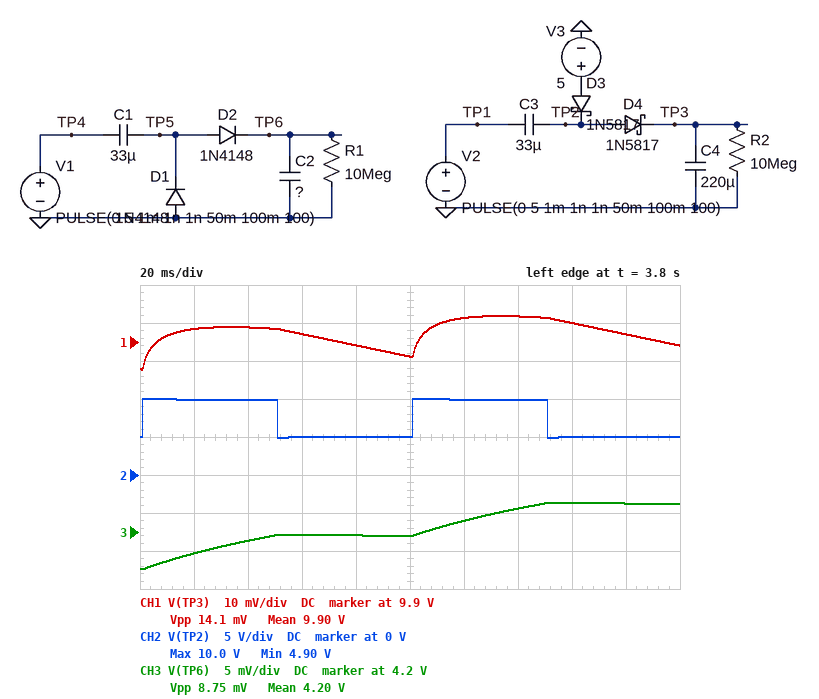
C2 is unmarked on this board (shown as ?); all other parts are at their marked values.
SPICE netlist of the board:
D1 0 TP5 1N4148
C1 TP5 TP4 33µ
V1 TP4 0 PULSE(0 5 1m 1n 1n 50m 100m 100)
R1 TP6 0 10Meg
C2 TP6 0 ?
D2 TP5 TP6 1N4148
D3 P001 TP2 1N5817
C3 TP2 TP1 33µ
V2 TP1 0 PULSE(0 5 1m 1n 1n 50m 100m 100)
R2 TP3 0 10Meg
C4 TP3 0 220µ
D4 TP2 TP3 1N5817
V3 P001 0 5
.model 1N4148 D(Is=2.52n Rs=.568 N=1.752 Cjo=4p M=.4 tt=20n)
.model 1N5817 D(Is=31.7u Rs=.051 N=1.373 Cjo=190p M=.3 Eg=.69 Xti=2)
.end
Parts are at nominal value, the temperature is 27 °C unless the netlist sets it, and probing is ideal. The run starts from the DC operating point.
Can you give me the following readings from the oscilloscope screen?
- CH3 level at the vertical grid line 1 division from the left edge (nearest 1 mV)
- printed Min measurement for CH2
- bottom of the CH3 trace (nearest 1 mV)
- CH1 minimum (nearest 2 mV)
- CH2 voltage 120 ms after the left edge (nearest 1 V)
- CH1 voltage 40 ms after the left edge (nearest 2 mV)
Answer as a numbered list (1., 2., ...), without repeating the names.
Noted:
1. 4.197 V
2. 4.90 V
3. 4.195 V
4. 9.892 V
5. 10 V
6. 9.904 V
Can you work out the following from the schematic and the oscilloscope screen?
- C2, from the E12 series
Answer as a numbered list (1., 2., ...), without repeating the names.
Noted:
1. 180 µF
